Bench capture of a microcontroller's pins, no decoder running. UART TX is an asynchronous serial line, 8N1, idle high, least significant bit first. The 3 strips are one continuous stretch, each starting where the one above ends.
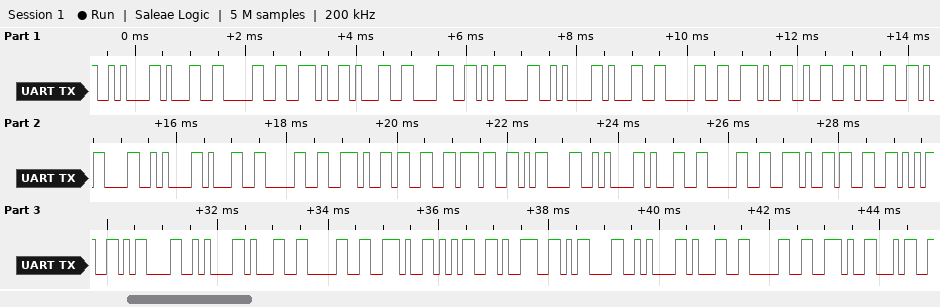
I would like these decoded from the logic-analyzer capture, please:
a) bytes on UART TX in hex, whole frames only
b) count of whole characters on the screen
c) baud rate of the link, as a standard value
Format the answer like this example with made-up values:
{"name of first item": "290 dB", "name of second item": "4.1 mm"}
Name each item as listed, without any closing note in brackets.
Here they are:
{"bytes on UART TX in hex, whole frames only": "0A 31 30 2E 31 38 0D 0A 31 30 2E 32 31 0D 0A 31 30 2E 33 37 0D 0A 31 30 2E 33 35 0D 0A 31 30 2E 35 39 0D 0A 31 30 2E 34", "count of whole characters on the screen": "40", "baud rate of the link, as a standard value": "9600 baud"}
